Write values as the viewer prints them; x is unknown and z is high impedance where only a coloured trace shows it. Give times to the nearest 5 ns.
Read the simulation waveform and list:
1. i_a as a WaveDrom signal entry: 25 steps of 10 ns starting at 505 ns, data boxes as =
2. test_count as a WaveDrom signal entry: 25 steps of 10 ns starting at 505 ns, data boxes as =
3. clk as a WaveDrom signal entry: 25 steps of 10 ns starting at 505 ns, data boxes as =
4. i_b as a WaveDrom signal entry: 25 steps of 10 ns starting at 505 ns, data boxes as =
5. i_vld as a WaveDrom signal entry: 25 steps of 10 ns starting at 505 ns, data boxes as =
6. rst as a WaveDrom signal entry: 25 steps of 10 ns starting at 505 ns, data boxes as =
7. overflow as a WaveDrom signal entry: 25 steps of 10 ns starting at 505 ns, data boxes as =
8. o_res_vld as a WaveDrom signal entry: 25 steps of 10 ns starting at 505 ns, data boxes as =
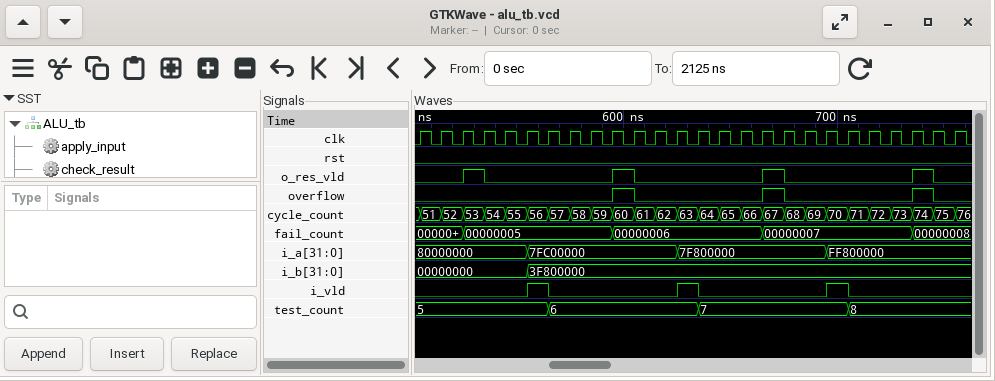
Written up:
{name: 'i_a', wave: '=....=......=......=.....', data: '80000000 7FC00000 7F800000 FF800000'}
{name: 'test_count', wave: '=.....=......=......=....', data: '5 6 7 8'}
{name: 'clk', wave: 'p........................'}
{name: 'i_b', wave: '=....=...................', data: '00000000 3F800000'}
{name: 'i_vld', wave: '0....10.....10.....10....'}
{name: 'rst', wave: '0........................'}
{name: 'overflow', wave: '0........10.....10.....10'}
{name: 'o_res_vld', wave: '0.10.....10.....10.....10'}
